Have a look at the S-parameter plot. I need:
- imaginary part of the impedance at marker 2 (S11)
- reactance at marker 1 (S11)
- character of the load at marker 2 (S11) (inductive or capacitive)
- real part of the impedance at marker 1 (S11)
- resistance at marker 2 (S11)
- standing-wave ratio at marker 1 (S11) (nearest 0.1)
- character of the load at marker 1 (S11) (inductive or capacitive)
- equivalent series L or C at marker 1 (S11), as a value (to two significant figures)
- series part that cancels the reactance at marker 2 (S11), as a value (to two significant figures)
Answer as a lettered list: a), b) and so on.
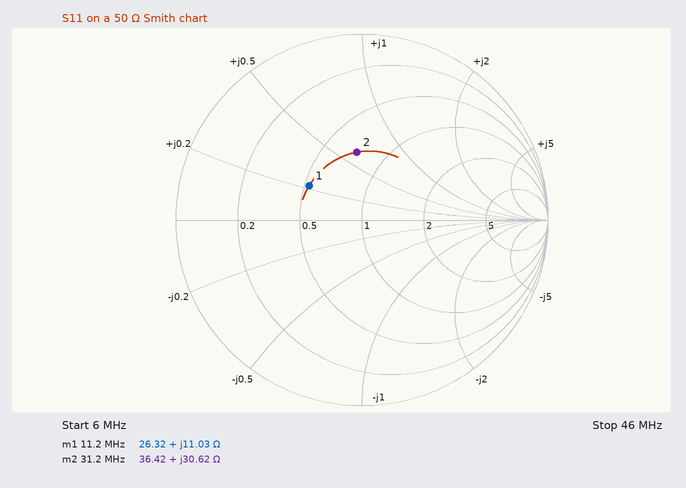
a) +30.62 Ω
b) +11.03 Ω
c) inductive
d) 26.32 Ω
e) 36.42 Ω
f) 2.0
g) inductive
h) 160 nH
i) 170 pF
